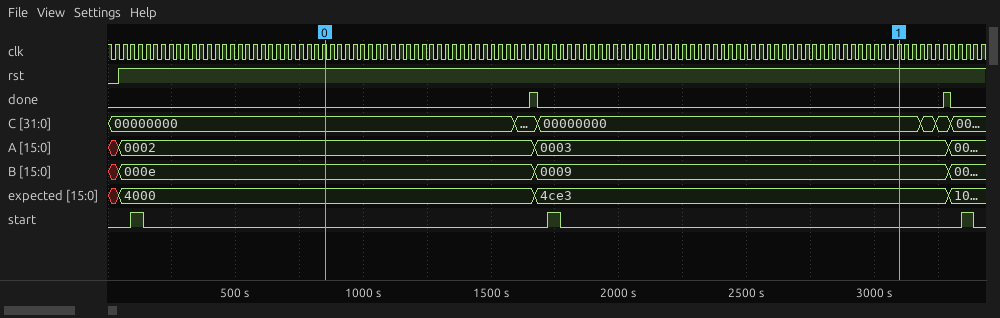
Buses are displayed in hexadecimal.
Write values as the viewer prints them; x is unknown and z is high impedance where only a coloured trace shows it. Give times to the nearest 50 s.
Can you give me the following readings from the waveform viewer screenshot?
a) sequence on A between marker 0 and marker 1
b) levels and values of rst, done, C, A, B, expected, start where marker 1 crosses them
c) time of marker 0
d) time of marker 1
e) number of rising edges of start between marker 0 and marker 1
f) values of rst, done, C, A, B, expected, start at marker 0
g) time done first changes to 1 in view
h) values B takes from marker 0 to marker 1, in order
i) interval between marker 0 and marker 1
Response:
0002, 0003
rst=1, done=0, C=00000000, A=0003, B=0009, expected=4ce3, start=0
850 s
3100 s
1
rst=1, done=0, C=00000000, A=0002, B=000e, expected=4000, start=0
1650 s
000e, 0009
2250 s
